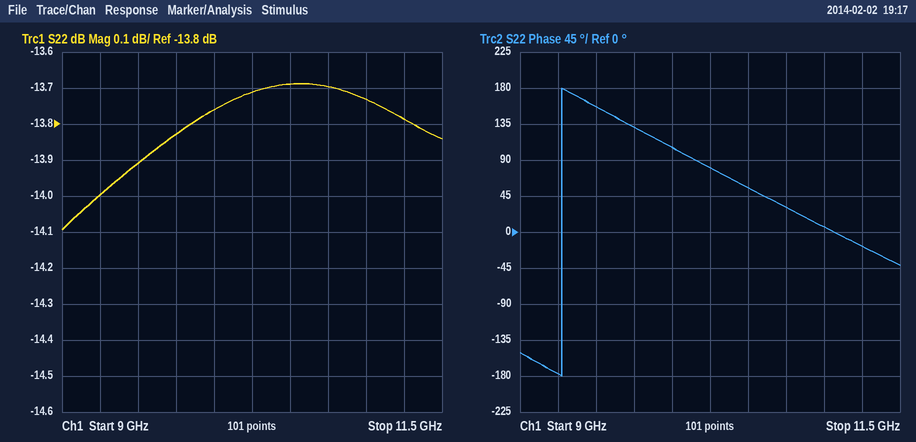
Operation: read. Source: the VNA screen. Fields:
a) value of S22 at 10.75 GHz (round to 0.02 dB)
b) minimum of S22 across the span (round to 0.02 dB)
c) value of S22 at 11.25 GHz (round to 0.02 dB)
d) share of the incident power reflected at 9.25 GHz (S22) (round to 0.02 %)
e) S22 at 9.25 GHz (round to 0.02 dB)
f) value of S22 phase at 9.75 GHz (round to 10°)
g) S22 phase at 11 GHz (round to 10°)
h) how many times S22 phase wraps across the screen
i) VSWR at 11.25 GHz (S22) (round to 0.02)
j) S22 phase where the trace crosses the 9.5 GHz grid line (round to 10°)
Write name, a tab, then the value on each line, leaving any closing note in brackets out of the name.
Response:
value of S22 at 10.75 GHz	-13.70 dB
minimum of S22 across the span	-14.10 dB
value of S22 at 11.25 GHz	-13.78 dB
share of the incident power reflected at 9.25 GHz (S22)	3.98 %
S22 at 9.25 GHz	-14.00 dB
value of S22 phase at 9.75 GHz	130°
S22 phase at 11 GHz	10°
how many times S22 phase wraps across the screen	1
VSWR at 11.25 GHz (S22)	1.52
S22 phase where the trace crosses the 9.5 GHz grid line	160°
